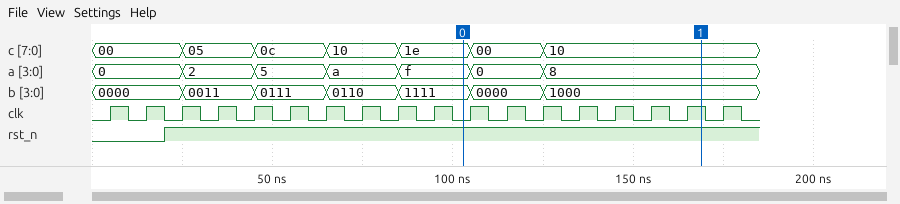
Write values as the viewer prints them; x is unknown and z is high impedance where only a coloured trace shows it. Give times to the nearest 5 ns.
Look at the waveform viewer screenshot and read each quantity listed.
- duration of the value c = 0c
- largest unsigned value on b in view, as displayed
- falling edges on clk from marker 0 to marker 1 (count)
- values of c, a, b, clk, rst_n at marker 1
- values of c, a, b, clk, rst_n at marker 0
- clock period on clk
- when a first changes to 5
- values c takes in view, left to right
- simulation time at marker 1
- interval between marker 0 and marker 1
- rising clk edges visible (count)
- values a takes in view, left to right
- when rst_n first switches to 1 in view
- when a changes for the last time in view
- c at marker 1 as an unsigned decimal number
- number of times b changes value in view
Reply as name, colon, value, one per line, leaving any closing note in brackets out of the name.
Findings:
duration of the value c = 0c: 20 ns
largest unsigned value on b in view, as displayed: 1111
falling edges on clk from marker 0 to marker 1: 6
values of c, a, b, clk, rst_n at marker 1: c=10, a=8, b=1000, clk=1, rst_n=1
values of c, a, b, clk, rst_n at marker 0: c=1e, a=f, b=1111, clk=0, rst_n=1
clock period on clk: 10 ns
when a first changes to 5: 45 ns
values c takes in view, left to right: 00, 05, 0c, 10, 1e, 00, 10
simulation time at marker 1: 170 ns
interval between marker 0 and marker 1: 65 ns
rising clk edges visible: 18
values a takes in view, left to right: 0, 2, 5, a, f, 0, 8
when rst_n first switches to 1 in view: 20 ns
when a changes for the last time in view: 125 ns
c at marker 1 as an unsigned decimal number: 16
number of times b changes value in view: 6
